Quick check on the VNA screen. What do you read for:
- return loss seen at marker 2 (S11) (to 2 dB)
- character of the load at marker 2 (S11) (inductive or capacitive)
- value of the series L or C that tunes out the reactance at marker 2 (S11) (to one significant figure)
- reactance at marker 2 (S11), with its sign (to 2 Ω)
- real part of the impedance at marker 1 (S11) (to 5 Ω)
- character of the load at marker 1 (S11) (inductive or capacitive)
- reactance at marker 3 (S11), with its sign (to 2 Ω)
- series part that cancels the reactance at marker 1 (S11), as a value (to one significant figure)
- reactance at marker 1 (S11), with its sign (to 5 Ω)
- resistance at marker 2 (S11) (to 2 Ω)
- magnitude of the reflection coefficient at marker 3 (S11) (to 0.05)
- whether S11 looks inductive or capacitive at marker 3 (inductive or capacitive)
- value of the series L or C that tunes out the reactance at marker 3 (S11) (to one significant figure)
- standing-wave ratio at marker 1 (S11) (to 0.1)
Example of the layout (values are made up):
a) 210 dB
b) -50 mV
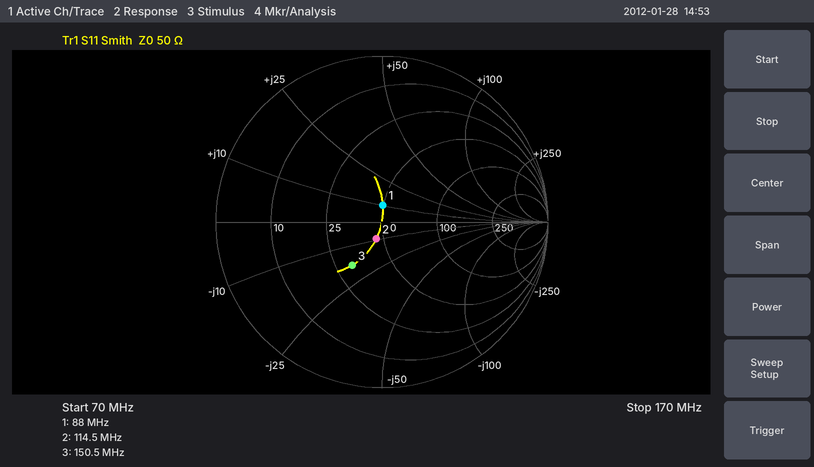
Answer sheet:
a) 20 dB
b) capacitive
c) 10 nH
d) -10 Ω
e) 50 Ω
f) inductive
g) -18 Ω
h) 200 pF
i) +10 Ω
j) 46 Ω
k) 0.30
l) capacitive
m) 20 nH
n) 1.2
